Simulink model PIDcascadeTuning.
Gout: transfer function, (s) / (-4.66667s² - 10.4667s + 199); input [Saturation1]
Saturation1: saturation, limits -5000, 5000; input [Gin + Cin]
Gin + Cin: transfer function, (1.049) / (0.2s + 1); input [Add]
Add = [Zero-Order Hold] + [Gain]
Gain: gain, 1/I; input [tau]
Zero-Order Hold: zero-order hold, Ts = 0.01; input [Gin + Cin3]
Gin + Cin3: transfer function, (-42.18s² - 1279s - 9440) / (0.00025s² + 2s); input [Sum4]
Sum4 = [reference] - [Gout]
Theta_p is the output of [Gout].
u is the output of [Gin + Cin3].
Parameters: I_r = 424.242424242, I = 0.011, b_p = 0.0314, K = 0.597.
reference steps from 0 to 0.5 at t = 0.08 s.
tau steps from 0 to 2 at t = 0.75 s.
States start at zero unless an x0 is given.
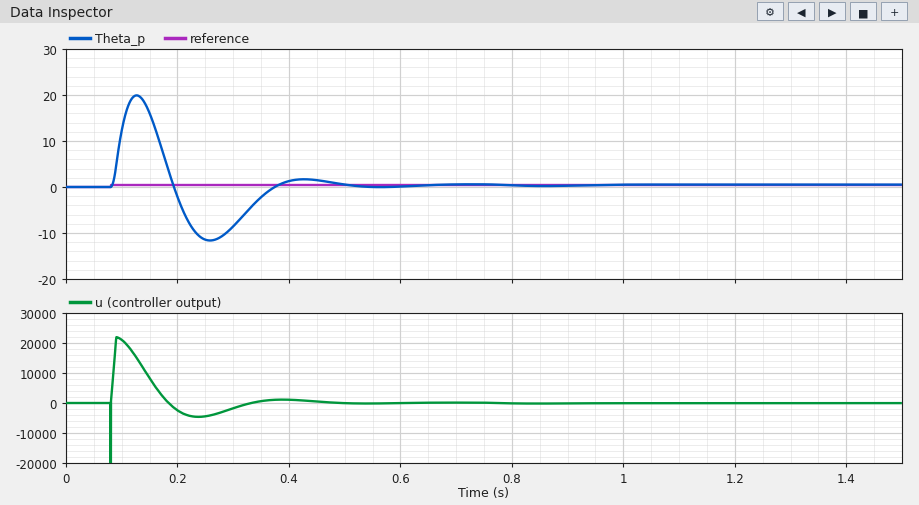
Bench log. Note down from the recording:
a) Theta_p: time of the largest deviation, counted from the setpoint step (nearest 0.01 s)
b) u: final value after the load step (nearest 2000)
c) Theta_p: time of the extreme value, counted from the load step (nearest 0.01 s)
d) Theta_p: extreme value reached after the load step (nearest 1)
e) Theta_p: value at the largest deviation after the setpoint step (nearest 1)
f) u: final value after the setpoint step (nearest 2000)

0.05 s
0
0.11 s
0
20
0
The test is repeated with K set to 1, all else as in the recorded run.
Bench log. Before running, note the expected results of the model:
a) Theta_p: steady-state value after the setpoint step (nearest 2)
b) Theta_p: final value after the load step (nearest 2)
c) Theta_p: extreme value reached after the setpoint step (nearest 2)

0
0
20
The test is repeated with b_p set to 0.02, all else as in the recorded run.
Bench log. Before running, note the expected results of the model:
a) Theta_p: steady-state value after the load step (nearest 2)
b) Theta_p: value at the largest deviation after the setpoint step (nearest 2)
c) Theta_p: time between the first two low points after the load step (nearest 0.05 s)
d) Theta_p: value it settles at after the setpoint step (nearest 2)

0
20
0.30 s
0
